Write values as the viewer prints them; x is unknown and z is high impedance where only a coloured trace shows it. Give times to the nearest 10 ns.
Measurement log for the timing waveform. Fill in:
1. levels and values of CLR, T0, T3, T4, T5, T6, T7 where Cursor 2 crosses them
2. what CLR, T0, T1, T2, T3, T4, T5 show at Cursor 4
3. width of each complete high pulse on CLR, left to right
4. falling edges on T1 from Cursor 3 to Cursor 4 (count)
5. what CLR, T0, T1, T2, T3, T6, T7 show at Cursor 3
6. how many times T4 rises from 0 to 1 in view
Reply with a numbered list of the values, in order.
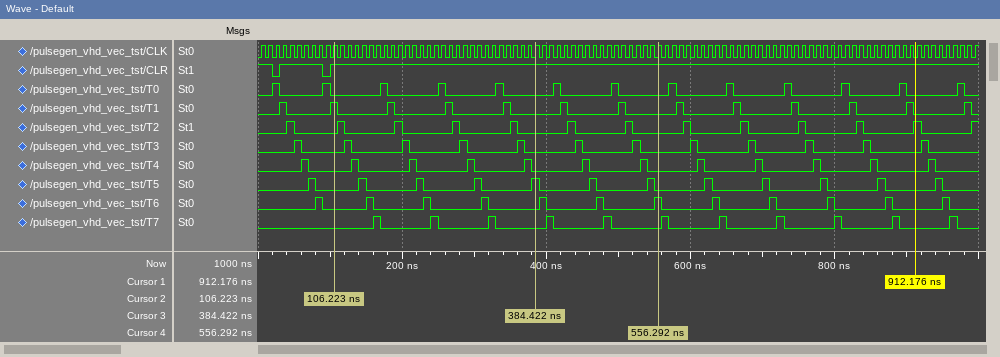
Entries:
1. CLR=1, T0=0, T3=0, T4=0, T5=0, T6=0, T7=0
2. CLR=1, T0=0, T1=0, T2=0, T3=0, T4=0, T5=0
3. 60 ns
4. 2
5. CLR=1, T0=0, T1=0, T2=0, T3=0, T6=0, T7=0
6. 12
